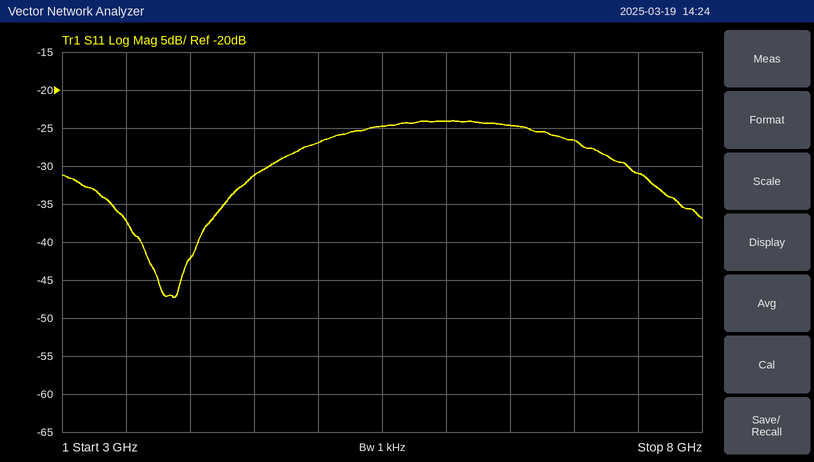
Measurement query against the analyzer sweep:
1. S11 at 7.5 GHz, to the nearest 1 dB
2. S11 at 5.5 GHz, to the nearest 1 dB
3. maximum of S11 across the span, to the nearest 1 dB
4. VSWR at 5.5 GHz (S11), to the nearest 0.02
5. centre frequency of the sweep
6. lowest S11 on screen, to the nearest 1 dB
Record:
-31 dB
-25 dB
-24 dB
1.12
5.5 GHz
-47 dB
